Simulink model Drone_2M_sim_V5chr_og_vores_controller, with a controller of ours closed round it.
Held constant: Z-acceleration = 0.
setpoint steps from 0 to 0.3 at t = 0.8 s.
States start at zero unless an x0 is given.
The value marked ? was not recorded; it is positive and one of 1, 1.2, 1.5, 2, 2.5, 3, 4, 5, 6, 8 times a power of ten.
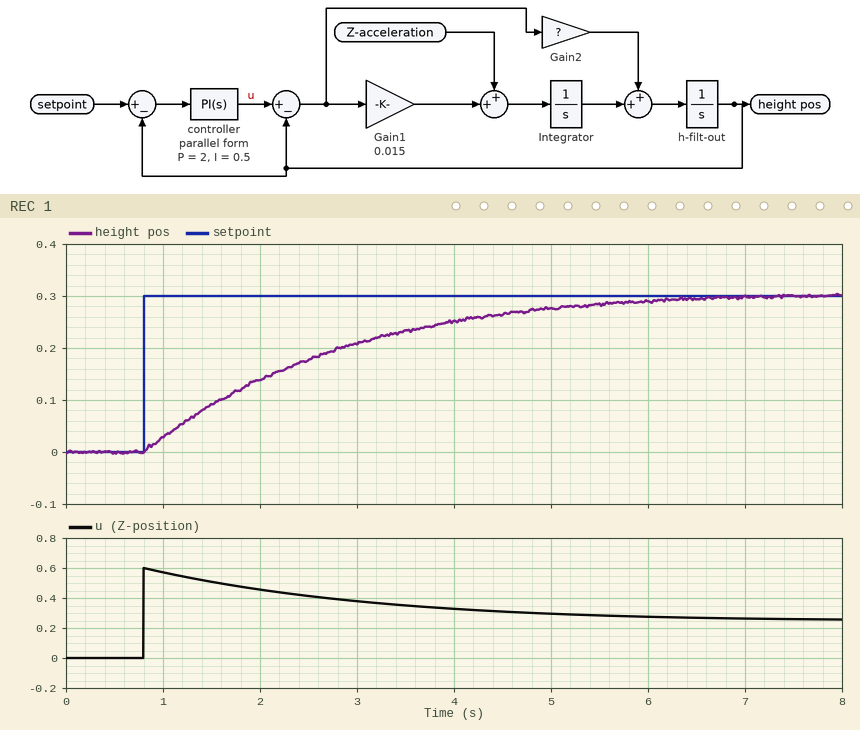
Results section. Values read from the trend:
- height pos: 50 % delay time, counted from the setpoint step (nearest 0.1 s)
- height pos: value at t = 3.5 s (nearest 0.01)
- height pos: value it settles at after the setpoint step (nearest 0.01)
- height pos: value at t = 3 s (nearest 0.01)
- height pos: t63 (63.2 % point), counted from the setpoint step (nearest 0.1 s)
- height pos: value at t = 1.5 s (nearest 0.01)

1.3 s
0.23
0.30
0.21
1.9 s
0.09
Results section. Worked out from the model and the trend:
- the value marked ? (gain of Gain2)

0.25
